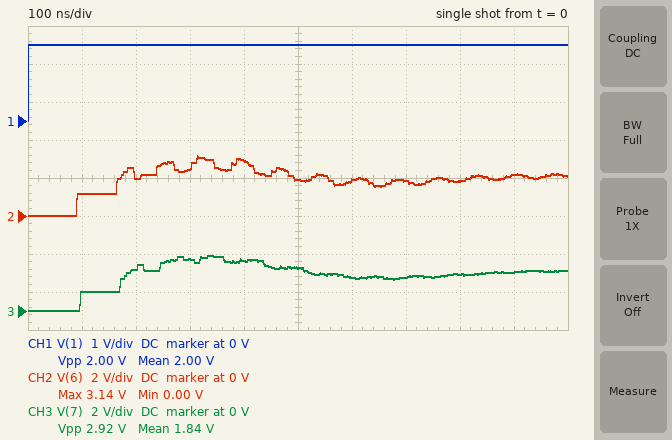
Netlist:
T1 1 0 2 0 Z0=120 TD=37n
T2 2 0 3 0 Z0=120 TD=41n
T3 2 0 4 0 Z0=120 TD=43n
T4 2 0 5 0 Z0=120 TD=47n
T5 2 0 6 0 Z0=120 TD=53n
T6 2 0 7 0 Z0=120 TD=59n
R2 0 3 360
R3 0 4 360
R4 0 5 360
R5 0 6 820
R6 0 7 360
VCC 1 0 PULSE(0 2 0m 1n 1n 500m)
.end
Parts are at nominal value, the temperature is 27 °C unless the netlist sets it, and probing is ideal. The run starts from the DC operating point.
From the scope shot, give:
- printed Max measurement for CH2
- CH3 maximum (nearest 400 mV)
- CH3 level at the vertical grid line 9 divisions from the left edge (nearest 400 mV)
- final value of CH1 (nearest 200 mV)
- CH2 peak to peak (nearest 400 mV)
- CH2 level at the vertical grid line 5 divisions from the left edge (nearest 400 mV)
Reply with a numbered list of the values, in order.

1. 3.14 V
2. 2.8 V
3. 2.0 V
4. 2.0 V
5. 3.2 V
6. 2.0 V
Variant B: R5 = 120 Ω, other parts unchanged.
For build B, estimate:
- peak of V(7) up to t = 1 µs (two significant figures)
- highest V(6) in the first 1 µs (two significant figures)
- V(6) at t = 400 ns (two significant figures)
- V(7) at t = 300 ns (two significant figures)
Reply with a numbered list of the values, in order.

1. 2.5 V
2. 2.4 V
3. 2.3 V
4. 2.1 V
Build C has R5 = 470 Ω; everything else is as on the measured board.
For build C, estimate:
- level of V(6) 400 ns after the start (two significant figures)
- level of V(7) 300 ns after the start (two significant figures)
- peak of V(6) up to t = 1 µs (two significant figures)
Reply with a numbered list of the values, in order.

1. 2.8 V
2. 2.6 V
3. 3.0 V
